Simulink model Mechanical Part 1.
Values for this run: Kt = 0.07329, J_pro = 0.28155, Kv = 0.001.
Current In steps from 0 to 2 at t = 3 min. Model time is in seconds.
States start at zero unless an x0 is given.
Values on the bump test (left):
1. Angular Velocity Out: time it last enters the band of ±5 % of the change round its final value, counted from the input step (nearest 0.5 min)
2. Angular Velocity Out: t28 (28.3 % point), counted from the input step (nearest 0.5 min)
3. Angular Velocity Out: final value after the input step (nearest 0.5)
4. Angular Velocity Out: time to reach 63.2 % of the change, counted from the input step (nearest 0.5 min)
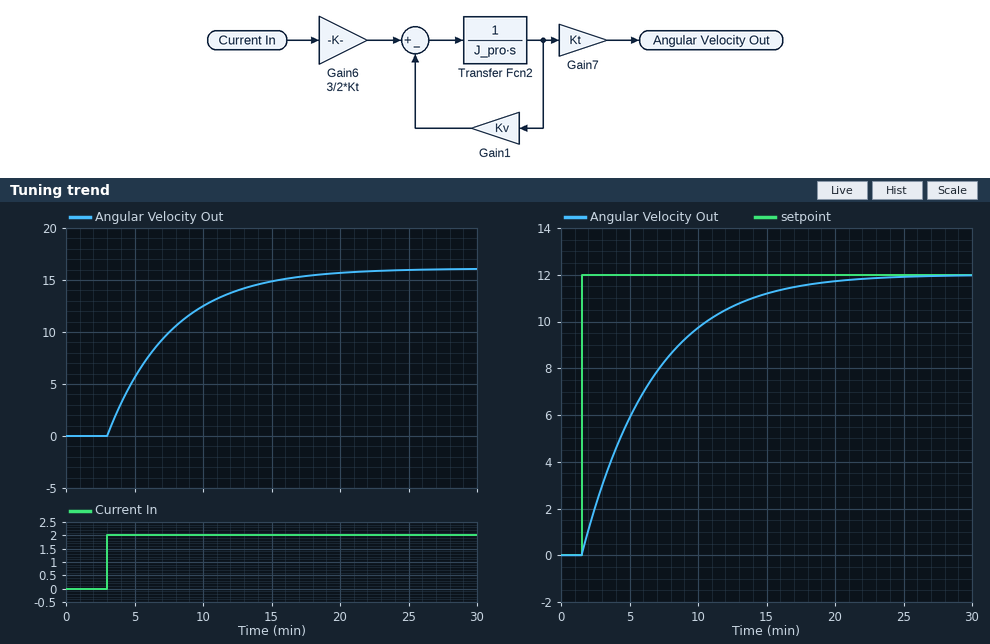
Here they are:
14.0 min
1.5 min
16.0
4.5 min
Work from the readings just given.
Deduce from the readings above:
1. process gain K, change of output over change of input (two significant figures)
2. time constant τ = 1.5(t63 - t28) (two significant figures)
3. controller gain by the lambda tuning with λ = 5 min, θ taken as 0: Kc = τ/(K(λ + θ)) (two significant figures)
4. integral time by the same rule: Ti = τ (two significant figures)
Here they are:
8.0
4.5 min
0.11
4.5 min
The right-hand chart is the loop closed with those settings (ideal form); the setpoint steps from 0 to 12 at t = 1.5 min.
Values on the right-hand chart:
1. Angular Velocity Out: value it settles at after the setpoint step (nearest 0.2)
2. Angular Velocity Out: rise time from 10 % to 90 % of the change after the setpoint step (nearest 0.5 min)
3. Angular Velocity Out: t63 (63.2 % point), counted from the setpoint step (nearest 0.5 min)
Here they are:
12.0
11.0 min
5.0 min
